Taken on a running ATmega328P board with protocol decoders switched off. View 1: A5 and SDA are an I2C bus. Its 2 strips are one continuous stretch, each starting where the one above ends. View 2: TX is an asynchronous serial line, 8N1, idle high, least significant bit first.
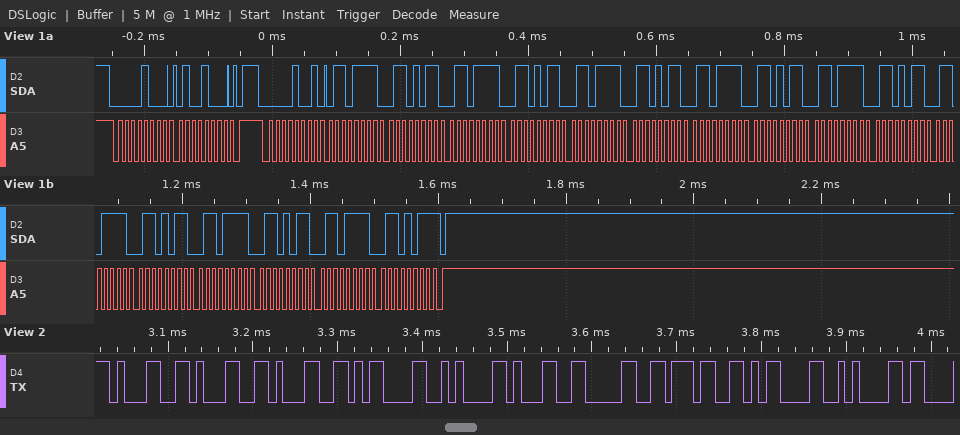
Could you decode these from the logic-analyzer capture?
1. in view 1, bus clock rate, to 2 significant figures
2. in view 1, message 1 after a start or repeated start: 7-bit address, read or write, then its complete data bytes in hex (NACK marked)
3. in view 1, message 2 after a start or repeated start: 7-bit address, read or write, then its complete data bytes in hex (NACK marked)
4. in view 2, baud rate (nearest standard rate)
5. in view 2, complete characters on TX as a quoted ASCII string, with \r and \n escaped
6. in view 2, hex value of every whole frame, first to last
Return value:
100 kHz
0x04 write: 48
0x04 read: 6F 6B 6F 6B 6F 6B 6F 6B 6F 6B 6F 6B 6F 6B 6F 6B NACK
115200 baud
"111\r\n107\r\n"
0x31 0x31 0x31 0x0D 0x0A 0x31 0x30 0x37 0x0D 0x0A
